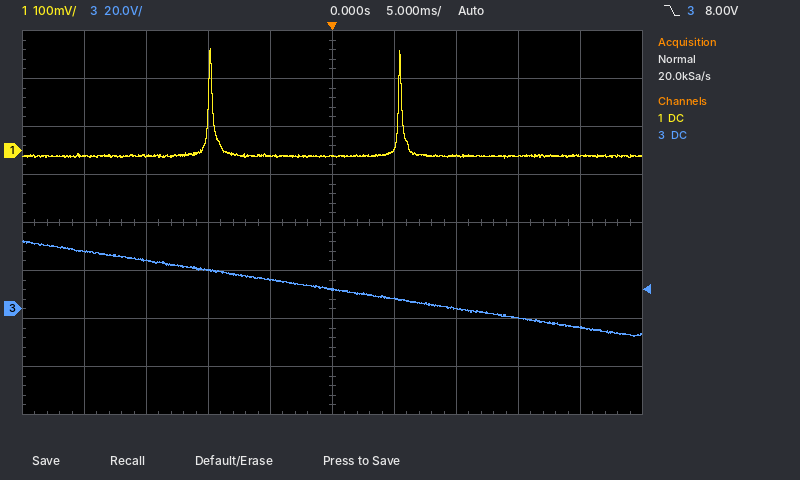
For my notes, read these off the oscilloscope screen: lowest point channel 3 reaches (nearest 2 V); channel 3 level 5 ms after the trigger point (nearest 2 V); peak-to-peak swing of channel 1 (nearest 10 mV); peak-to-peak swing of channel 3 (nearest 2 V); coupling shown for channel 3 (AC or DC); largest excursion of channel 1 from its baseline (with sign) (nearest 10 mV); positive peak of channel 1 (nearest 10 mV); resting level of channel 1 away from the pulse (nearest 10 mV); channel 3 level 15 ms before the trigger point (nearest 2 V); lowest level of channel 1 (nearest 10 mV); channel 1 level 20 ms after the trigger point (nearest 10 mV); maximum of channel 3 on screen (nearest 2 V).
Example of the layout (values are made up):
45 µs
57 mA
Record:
-12 V
4 V
230 mV
40 V
DC
+220 mV
210 mV
-10 mV
20 V
-20 mV
-10 mV
28 V
